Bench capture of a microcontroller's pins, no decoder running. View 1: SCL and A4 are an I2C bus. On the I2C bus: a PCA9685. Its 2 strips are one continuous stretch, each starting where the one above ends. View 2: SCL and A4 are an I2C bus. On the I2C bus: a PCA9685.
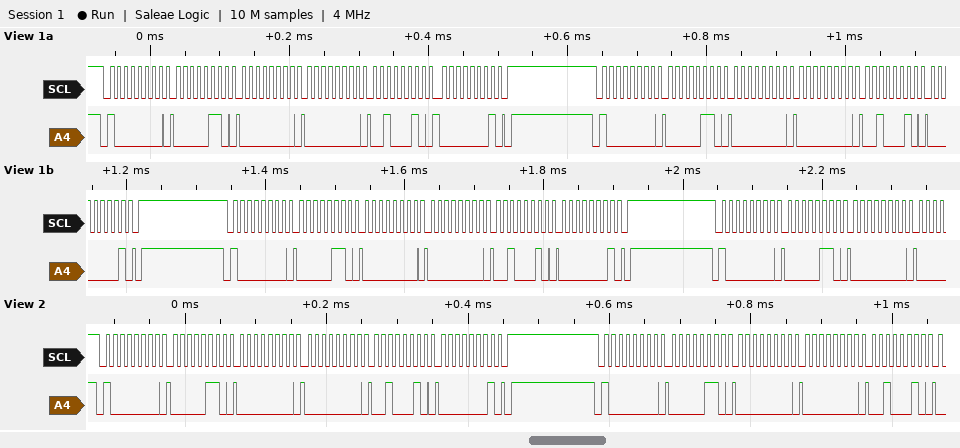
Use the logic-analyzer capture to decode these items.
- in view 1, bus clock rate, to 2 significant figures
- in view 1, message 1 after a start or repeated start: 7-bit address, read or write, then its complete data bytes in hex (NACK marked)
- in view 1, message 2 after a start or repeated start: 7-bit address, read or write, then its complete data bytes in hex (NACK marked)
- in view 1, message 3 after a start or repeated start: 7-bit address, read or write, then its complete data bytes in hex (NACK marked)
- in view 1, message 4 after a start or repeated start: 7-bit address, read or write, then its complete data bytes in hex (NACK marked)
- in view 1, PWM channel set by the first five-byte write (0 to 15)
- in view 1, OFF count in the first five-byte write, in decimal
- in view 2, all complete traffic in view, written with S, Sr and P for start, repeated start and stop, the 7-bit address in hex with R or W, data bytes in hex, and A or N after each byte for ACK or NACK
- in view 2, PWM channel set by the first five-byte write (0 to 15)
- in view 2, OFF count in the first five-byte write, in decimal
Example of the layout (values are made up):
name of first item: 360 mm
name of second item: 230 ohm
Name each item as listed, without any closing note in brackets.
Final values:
in view 1, bus clock rate, to 2 significant figures: 100 kHz
in view 1, message 1 after a start or repeated start: 7-bit address, read or write, then its complete data bytes in hex: 0x40 write: 06 00 00 22 01
in view 1, message 2 after a start or repeated start: 7-bit address, read or write, then its complete data bytes in hex: 0x40 write: 06 00 00 22 01
in view 1, message 3 after a start or repeated start: 7-bit address, read or write, then its complete data bytes in hex: 0x40 write: 06 00 00 22 01
in view 1, message 4 after a start or repeated start: 7-bit address, read or write, then its complete data bytes in hex: 0x40 write: 06 00
in view 1, PWM channel set by the first five-byte write: 0
in view 1, OFF count in the first five-byte write, in decimal: 290
in view 2, all complete traffic in view, written with S, Sr and P for start, repeated start and stop, the 7-bit address in hex with R or W, data bytes in hex, and A or N after each byte for ACK or NACK: S 40W A 06 A 00 A 00 A 22 A 01 A P S 40W A 06 A 00 A 00 A 22 A
in view 2, PWM channel set by the first five-byte write: 0
in view 2, OFF count in the first five-byte write, in decimal: 290
